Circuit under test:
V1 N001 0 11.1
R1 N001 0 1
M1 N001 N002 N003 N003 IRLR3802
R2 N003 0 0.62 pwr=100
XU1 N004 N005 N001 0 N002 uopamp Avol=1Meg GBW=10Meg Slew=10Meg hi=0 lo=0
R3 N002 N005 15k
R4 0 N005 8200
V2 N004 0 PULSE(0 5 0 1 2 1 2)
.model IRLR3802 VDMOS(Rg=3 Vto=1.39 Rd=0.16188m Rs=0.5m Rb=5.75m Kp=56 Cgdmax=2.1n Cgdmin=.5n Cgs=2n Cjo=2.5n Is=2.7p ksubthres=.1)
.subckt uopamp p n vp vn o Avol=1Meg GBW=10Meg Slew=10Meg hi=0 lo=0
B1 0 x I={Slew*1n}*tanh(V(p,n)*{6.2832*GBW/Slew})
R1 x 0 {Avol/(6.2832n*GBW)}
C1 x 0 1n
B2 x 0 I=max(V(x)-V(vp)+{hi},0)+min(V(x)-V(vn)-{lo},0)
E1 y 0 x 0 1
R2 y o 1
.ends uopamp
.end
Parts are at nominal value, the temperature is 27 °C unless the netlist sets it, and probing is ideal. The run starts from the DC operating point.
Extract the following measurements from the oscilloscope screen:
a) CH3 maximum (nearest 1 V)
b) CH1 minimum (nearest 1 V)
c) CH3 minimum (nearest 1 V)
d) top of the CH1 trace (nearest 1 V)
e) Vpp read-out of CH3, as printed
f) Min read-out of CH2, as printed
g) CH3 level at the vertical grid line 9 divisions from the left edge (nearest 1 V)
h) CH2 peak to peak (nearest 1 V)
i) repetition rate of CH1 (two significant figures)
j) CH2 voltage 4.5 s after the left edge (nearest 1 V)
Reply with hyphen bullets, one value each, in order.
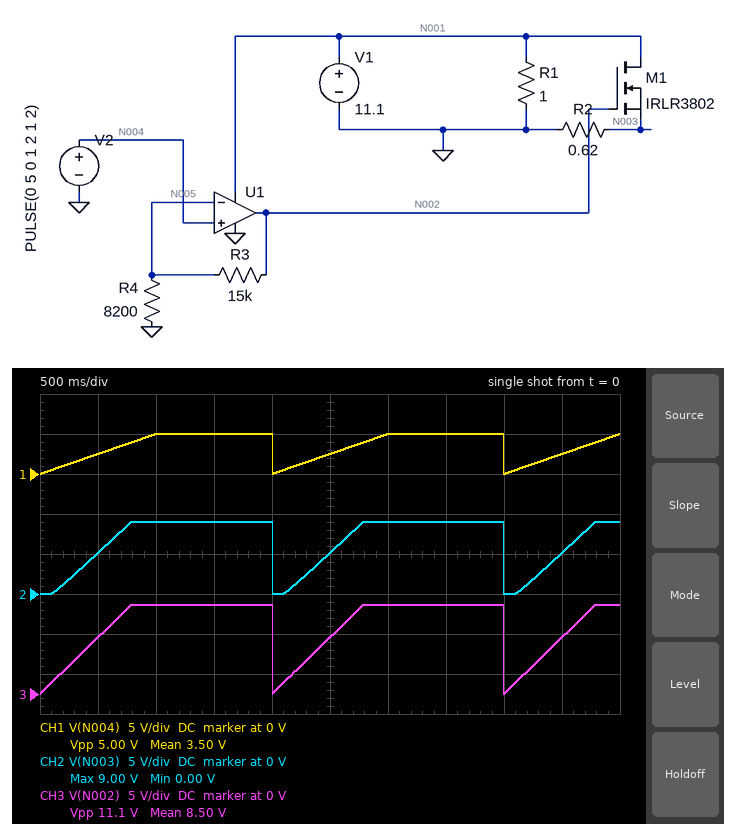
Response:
- 11 V
- 0 V
- 0 V
- 5 V
- 11.1 V
- 0.00 V
- 7 V
- 9 V
- 500 mHz
- 5 V
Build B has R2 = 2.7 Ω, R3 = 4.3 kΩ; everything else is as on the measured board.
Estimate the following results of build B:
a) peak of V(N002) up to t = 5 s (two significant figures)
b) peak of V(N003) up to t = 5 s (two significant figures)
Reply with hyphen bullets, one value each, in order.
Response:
- 7.6 V
- 6.0 V
